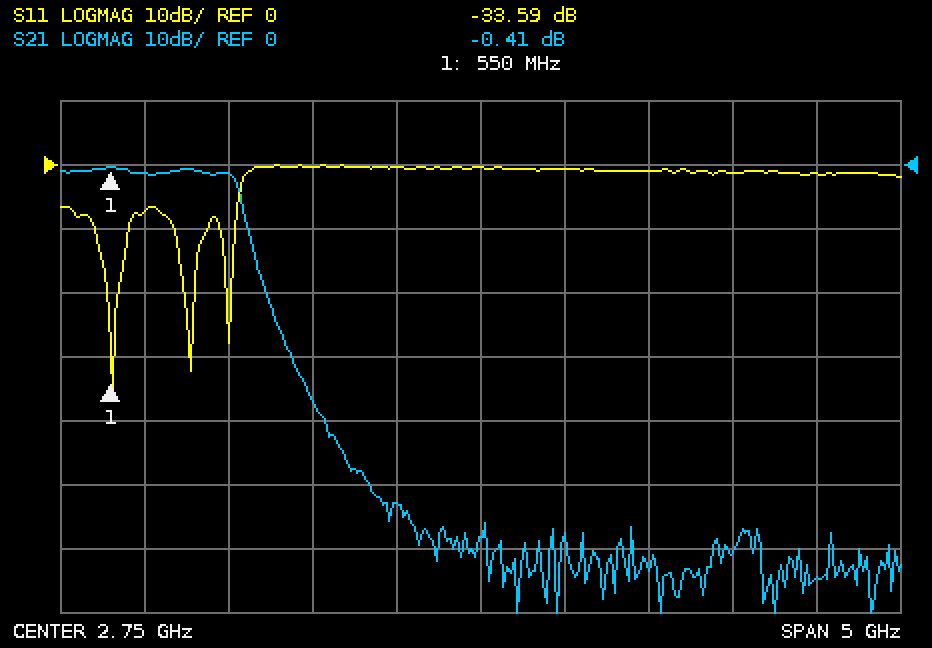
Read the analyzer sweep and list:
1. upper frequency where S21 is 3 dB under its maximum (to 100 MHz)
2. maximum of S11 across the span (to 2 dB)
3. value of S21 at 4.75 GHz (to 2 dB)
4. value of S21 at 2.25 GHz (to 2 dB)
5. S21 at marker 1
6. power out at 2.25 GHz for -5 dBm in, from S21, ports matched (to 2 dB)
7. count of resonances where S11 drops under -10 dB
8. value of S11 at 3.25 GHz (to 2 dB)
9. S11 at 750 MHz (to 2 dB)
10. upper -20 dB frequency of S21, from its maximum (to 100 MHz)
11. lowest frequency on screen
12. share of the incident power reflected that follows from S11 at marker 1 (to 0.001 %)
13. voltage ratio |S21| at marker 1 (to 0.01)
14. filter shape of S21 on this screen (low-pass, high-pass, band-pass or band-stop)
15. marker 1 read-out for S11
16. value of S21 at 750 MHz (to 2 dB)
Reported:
1.3 GHz
0 dB
-64 dB
-52 dB
-0.41 dB
-58 dBm
3
0 dB
-8 dB
1.5 GHz
250 MHz
0.044 %
0.95
low-pass
-33.59 dB
-2 dB
